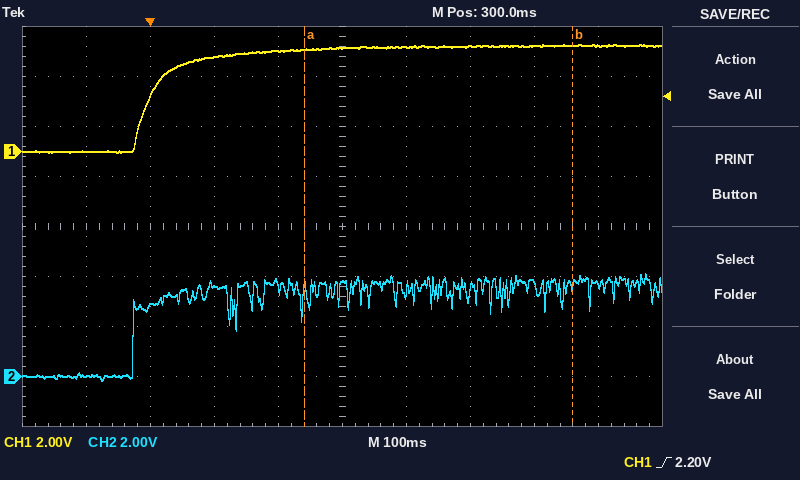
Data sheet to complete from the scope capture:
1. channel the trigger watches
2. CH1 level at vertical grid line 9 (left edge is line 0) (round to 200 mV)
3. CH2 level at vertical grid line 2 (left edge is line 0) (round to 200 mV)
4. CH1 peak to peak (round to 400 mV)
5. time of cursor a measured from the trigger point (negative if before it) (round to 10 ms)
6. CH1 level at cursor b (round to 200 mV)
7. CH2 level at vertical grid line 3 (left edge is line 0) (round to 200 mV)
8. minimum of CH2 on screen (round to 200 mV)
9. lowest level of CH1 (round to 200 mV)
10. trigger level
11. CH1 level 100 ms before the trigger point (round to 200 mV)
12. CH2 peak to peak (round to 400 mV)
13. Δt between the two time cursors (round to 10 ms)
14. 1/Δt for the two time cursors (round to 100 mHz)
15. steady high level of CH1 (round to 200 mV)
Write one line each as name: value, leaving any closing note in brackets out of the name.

channel the trigger watches: CH1
CH1 level at vertical grid line 9 (left edge is line 0): 4.2 V
CH2 level at vertical grid line 2 (left edge is line 0): 2.8 V
CH1 peak to peak: 4.4 V
time of cursor a measured from the trigger point (negative if before it): +240 ms
CH1 level at cursor b: 4.2 V
CH2 level at vertical grid line 3 (left edge is line 0): 3.6 V
minimum of CH2 on screen: -200 mV
lowest level of CH1: 0.0 V
trigger level: 2.20 V
CH1 level 100 ms before the trigger point: 0.0 V
CH2 peak to peak: 4.4 V
Δt between the two time cursors: 420 ms
1/Δt for the two time cursors: 2.4 Hz
steady high level of CH1: 4.2 V
